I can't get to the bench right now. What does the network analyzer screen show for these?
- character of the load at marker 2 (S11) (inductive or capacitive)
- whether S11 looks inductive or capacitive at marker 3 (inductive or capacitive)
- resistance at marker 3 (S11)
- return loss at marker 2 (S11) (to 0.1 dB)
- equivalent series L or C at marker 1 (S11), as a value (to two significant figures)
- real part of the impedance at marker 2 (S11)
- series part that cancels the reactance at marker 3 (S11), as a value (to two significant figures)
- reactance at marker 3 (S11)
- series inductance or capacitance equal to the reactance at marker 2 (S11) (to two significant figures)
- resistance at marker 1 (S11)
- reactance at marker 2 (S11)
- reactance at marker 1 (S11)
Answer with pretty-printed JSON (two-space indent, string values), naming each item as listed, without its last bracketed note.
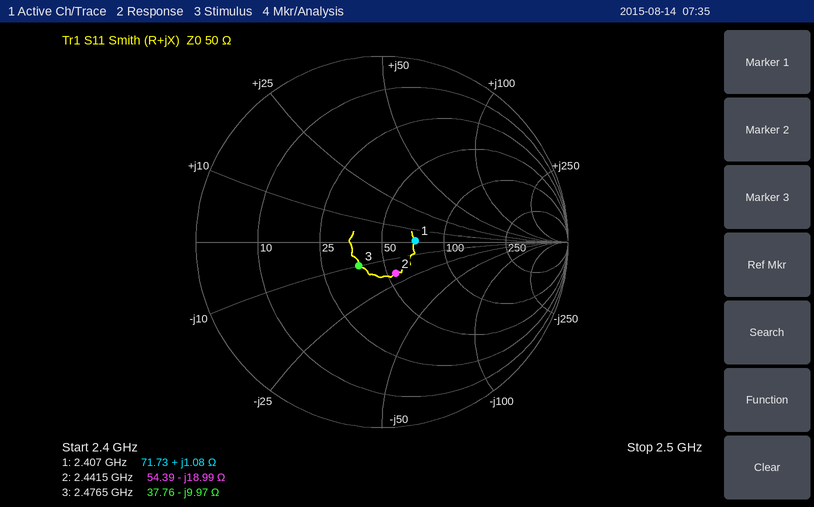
{
  "character of the load at marker 2 (S11)": "capacitive",
  "whether S11 looks inductive or capacitive at marker 3": "capacitive",
  "resistance at marker 3": "37.76 Ω",
  "return loss at marker 2 (S11)": "14.7 dB",
  "equivalent series L or C at marker 1 (S11), as a value": "71 pH",
  "real part of the impedance at marker 2": "54.39 Ω",
  "series part that cancels the reactance at marker 3 (S11), as a value": "640 pH",
  "reactance at marker 3": "-9.97 Ω",
  "series inductance or capacitance equal to the reactance at marker 2 (S11)": "3.4 pF",
  "resistance at marker 1": "71.73 Ω",
  "reactance at marker 2": "-18.99 Ω",
  "reactance at marker 1": "+1.08 Ω"
}
